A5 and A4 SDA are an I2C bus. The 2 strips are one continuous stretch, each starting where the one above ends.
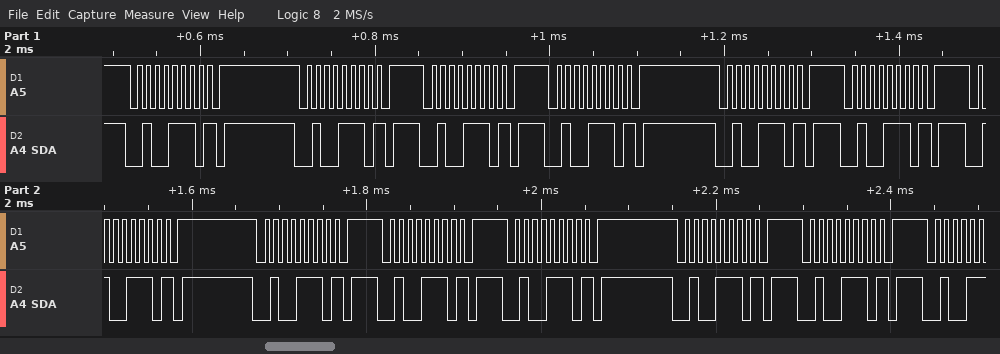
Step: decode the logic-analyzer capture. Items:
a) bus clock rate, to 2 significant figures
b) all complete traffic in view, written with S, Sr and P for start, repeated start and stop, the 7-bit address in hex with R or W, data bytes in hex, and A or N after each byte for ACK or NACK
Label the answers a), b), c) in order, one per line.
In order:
a) 100 kHz
b) S 27W N P S 27W N P S 27W N P S 27W N P S 27W N P S 27W N P S 27W N P S 27W N P S 27W N P S 27W N P S 27W N P S 27W N P
